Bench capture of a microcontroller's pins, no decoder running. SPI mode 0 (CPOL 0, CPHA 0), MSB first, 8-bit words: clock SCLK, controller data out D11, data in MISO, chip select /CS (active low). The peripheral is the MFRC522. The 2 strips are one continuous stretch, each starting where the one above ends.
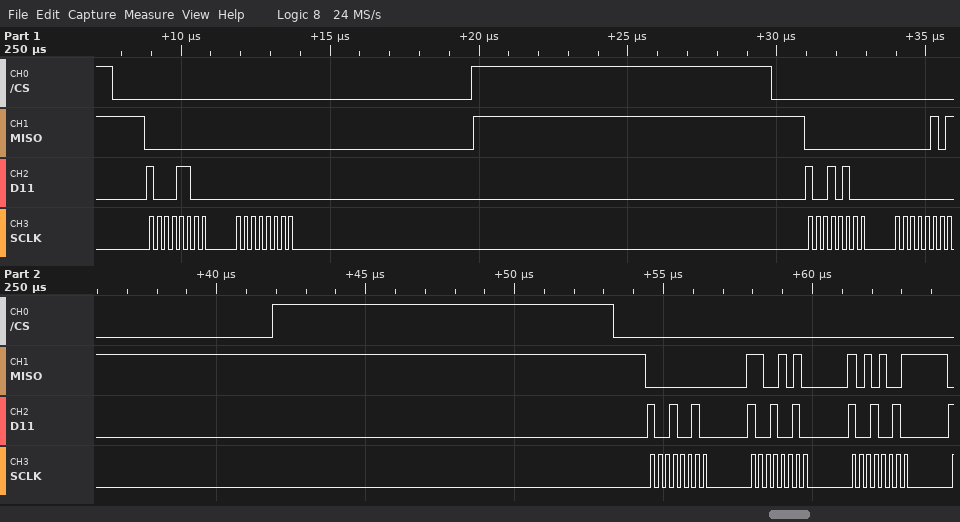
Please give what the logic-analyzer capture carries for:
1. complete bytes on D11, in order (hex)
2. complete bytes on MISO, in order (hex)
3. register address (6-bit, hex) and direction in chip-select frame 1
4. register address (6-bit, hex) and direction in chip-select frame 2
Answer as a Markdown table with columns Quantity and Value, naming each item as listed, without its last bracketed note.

| Quantity | Value |
|---|---|
| complete bytes on D11, in order | 0x8C 0x00 0x94 0x00 0x92 0x92 0x92 |
| complete bytes on MISO, in order | 0x00 0x00 0x00 0x05 0x00 0xCA 0xA9 |
| register address (6-bit, hex) and direction in chip-select frame 1 | 0x06 read |
| register address (6-bit, hex) and direction in chip-select frame 2 | 0x0A read |
